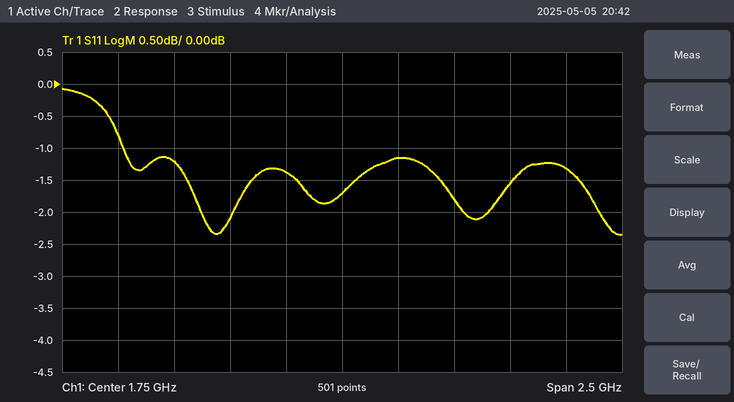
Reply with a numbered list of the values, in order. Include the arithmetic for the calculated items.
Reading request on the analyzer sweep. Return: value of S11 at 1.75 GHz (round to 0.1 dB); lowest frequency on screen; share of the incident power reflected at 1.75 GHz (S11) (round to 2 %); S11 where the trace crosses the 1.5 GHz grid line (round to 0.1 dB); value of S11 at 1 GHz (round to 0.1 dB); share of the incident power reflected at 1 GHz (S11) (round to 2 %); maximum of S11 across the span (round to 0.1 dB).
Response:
1. -1.7 dB
2. 500 MHz
3. 10^(-1.7/10) ≈ 68 %
4. -1.4 dB
5. -1.2 dB
6. 10^(-1.2/10) ≈ 76 %
7. -0.1 dB
